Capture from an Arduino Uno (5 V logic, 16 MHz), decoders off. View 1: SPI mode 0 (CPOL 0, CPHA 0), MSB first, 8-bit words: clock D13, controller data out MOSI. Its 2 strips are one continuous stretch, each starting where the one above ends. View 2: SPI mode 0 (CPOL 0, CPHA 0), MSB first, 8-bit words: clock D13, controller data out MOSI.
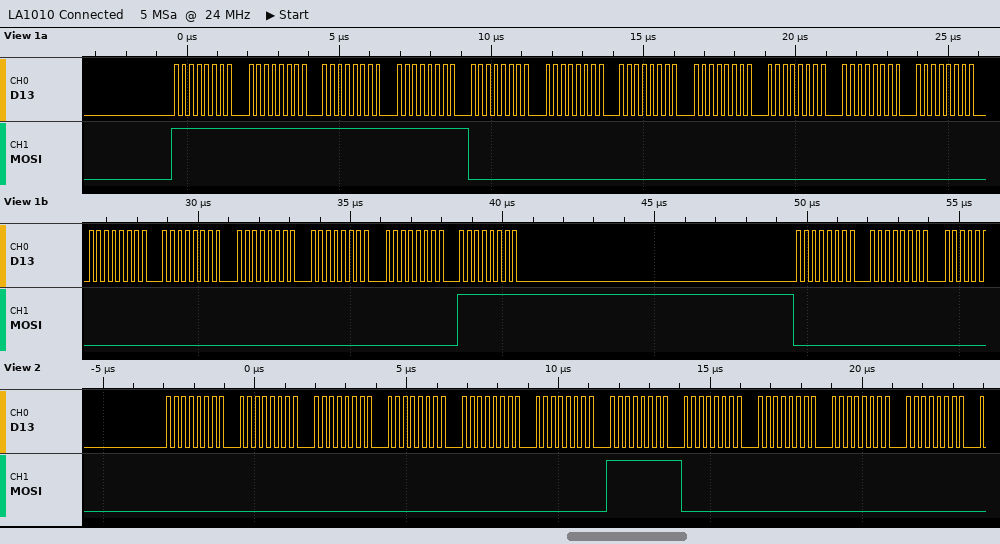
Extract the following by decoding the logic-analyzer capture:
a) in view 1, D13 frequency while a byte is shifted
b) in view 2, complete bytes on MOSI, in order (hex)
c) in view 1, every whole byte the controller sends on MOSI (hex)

4 MHz
0x00 0x00 0x00 0x00 0x00 0x00 0xFF 0x00 0x00 0x00 0x00
0xFF 0xFF 0xFF 0xFF 0x00 0x00 0x00 0x00 0x00 0x00 0x00 0x00 0x00 0x00 0x00 0x00 0xFF 0x00 0x00
